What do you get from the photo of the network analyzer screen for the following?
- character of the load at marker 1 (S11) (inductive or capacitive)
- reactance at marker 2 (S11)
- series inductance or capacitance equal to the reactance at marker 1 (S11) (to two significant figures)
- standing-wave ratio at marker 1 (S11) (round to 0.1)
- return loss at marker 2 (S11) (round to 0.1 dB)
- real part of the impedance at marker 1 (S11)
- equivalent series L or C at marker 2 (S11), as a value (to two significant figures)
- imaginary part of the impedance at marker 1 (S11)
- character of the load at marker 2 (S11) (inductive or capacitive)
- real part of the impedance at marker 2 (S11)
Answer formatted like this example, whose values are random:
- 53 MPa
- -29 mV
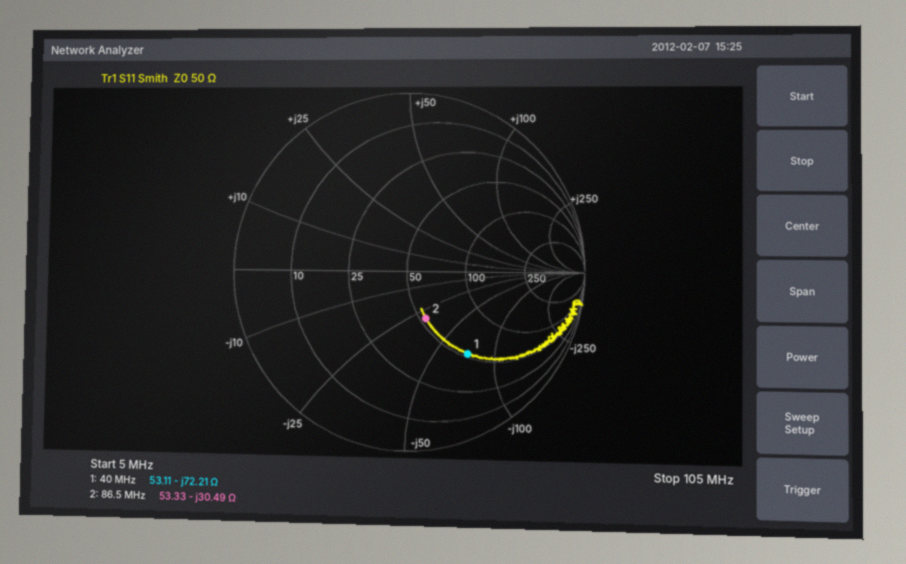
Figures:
- capacitive
- -30.49 Ω
- 55 pF
- 3.7
- 10.9 dB
- 53.11 Ω
- 60 pF
- -72.21 Ω
- capacitive
- 53.33 Ω
